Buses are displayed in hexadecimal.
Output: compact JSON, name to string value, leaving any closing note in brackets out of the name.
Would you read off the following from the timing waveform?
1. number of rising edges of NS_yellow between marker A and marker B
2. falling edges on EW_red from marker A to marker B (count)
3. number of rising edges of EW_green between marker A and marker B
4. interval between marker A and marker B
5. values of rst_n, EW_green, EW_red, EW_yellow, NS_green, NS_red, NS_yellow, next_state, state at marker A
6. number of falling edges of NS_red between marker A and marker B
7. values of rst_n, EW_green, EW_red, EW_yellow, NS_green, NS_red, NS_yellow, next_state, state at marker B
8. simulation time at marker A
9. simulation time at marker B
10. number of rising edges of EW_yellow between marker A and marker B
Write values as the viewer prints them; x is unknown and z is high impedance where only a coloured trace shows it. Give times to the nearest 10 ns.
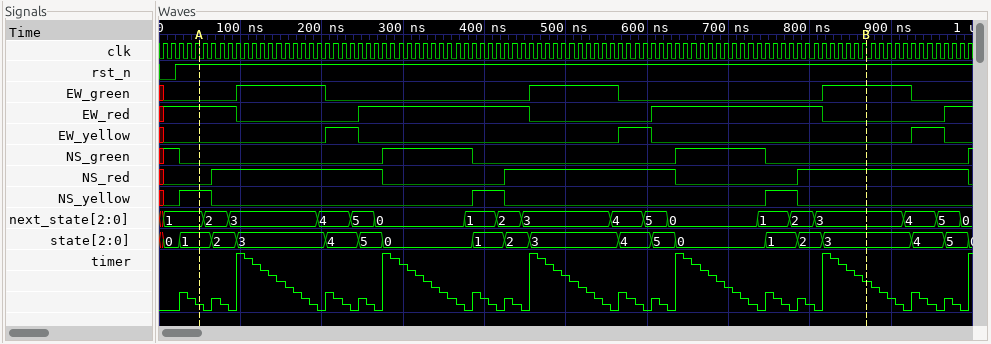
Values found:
{"number of rising edges of NS_yellow between marker A and marker B": "2", "falling edges on EW_red from marker A to marker B": "3", "number of rising edges of EW_green between marker A and marker B": "3", "interval between marker A and marker B": "820 ns", "values of rst_n, EW_green, EW_red, EW_yellow, NS_green, NS_red, NS_yellow, next_state, state at marker A": "rst_n=1, EW_green=0, EW_red=1, EW_yellow=0, NS_green=0, NS_red=0, NS_yellow=1, next_state=1, state=1", "number of falling edges of NS_red between marker A and marker B": "2", "values of rst_n, EW_green, EW_red, EW_yellow, NS_green, NS_red, NS_yellow, next_state, state at marker B": "rst_n=1, EW_green=1, EW_red=0, EW_yellow=0, NS_green=0, NS_red=1, NS_yellow=0, next_state=3, state=3", "simulation time at marker A": "50 ns", "simulation time at marker B": "870 ns", "number of rising edges of EW_yellow between marker A and marker B": "2"}
